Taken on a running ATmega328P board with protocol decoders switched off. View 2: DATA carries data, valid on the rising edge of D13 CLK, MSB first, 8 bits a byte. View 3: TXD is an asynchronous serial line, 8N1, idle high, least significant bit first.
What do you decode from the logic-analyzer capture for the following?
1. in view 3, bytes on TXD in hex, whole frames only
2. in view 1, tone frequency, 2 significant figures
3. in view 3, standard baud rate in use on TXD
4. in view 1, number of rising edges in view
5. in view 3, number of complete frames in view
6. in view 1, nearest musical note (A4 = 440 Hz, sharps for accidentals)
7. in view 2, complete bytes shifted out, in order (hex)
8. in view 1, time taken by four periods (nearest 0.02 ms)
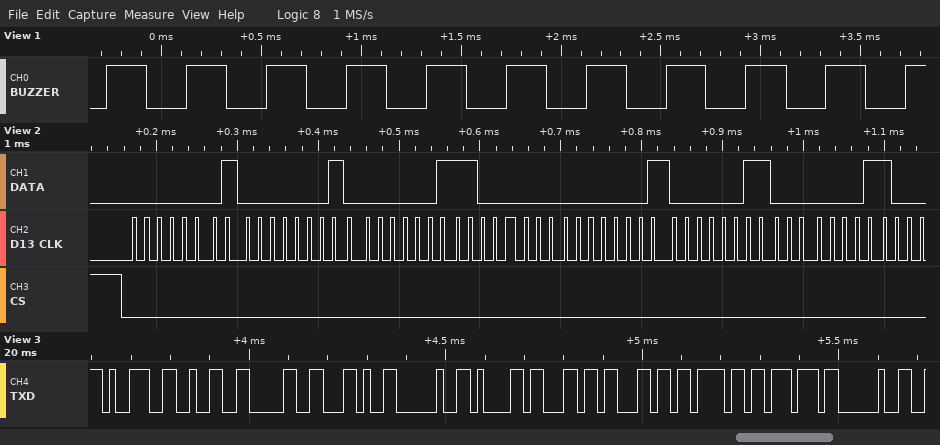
39 32 30 2C 20 61 6C 6C 6F 77 20
2.5 kHz
57600 baud
11
11
D#7
0x01 0x01 0x01 0xC0 0x01 0x03 0x01
1.60 ms
